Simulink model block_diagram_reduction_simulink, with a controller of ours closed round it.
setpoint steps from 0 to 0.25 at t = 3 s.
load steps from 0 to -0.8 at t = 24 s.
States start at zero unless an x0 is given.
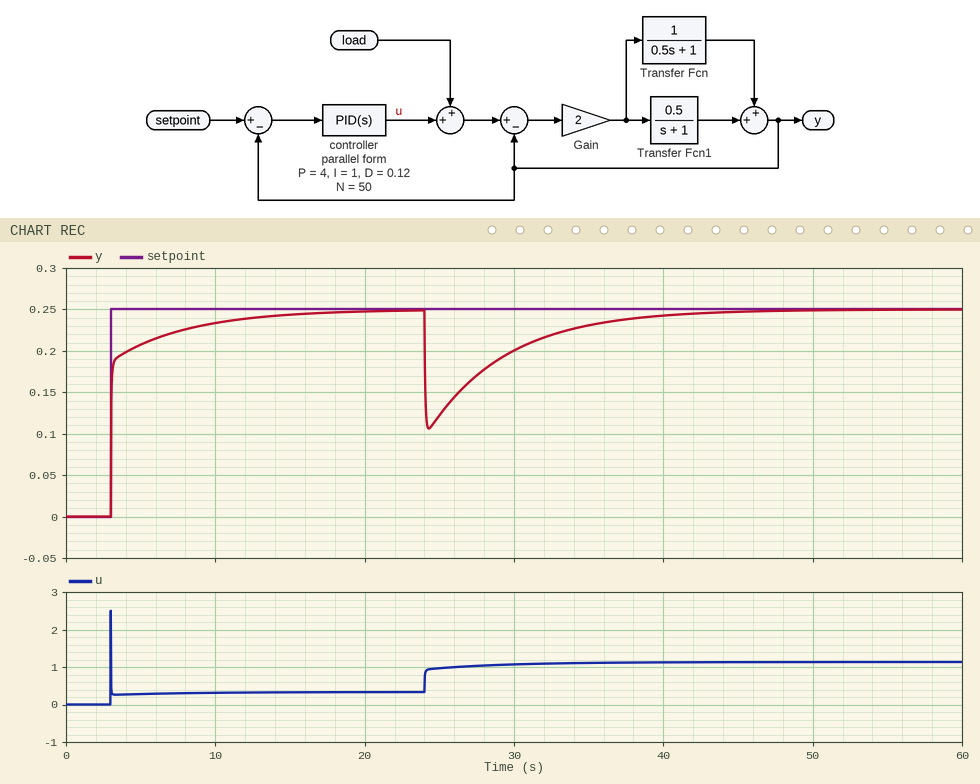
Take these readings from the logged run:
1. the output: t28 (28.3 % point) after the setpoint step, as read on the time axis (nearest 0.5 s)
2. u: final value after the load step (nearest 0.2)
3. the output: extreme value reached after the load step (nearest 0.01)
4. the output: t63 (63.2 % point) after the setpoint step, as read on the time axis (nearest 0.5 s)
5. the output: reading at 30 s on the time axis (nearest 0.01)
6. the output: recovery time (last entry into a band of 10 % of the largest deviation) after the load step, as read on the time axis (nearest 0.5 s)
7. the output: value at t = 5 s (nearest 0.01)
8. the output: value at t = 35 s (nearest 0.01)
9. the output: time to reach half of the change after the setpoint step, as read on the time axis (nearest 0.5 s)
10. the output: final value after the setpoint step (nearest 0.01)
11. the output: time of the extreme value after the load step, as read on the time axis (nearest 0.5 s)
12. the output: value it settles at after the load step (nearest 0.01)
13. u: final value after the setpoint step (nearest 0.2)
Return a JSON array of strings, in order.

["3.0 s", "1.2", "0.11", "3.0 s", "0.20", "36.5 s", "0.21", "0.23", "3.0 s", "0.25", "24.5 s", "0.25", "0.4"]
